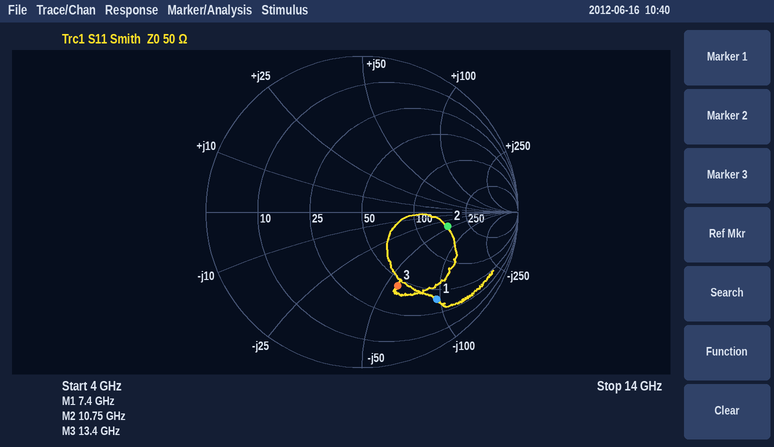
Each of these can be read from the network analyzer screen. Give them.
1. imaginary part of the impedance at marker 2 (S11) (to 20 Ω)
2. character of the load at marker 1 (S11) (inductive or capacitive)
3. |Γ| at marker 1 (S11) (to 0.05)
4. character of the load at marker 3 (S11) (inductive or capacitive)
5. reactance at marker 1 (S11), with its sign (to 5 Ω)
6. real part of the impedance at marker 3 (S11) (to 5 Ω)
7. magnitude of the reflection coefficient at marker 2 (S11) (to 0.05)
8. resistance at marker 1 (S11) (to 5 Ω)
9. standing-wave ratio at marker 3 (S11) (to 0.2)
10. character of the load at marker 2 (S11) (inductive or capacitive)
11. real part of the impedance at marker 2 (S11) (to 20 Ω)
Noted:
-40 Ω
capacitive
0.75
capacitive
-95 Ω
45 Ω
0.55
40 Ω
3.2
capacitive
160 Ω
